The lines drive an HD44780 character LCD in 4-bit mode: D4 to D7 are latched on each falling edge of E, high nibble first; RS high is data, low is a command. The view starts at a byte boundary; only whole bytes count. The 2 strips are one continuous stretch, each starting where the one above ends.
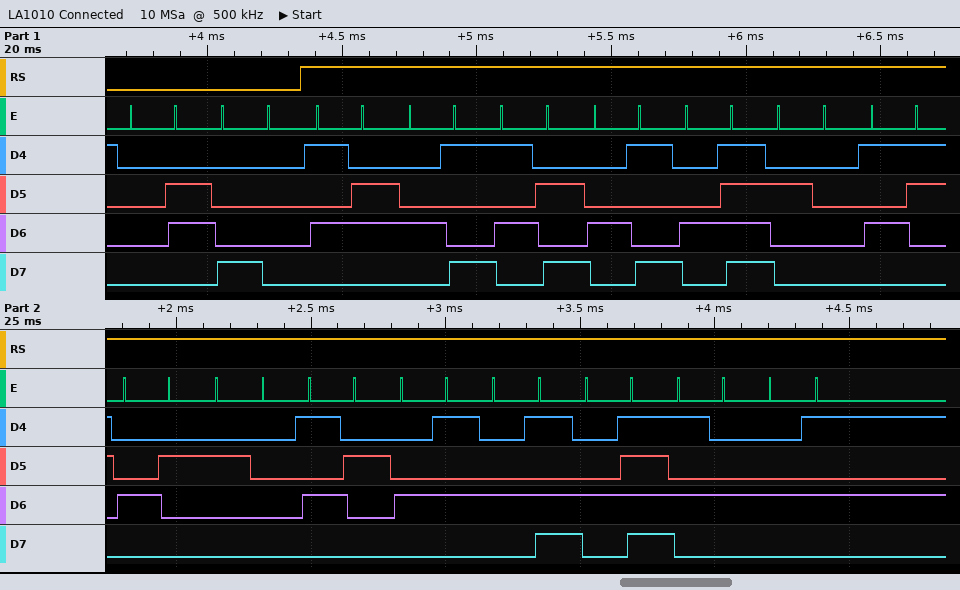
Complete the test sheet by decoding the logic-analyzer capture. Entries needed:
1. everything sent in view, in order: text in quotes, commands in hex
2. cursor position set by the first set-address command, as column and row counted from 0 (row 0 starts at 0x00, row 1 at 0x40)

0x06 0x80 "VIZIO SB REMOTE"
column 0, row 0
